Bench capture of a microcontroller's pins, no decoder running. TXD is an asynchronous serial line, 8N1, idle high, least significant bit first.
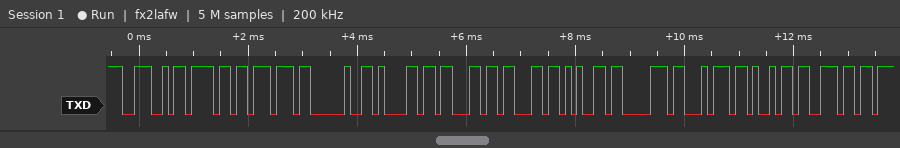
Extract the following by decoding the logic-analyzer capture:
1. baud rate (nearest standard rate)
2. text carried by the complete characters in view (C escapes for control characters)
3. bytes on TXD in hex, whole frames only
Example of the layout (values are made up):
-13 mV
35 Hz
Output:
9600 baud
"Now acceptin"
4E 6F 77 20 61 63 63 65 70 74 69 6E
